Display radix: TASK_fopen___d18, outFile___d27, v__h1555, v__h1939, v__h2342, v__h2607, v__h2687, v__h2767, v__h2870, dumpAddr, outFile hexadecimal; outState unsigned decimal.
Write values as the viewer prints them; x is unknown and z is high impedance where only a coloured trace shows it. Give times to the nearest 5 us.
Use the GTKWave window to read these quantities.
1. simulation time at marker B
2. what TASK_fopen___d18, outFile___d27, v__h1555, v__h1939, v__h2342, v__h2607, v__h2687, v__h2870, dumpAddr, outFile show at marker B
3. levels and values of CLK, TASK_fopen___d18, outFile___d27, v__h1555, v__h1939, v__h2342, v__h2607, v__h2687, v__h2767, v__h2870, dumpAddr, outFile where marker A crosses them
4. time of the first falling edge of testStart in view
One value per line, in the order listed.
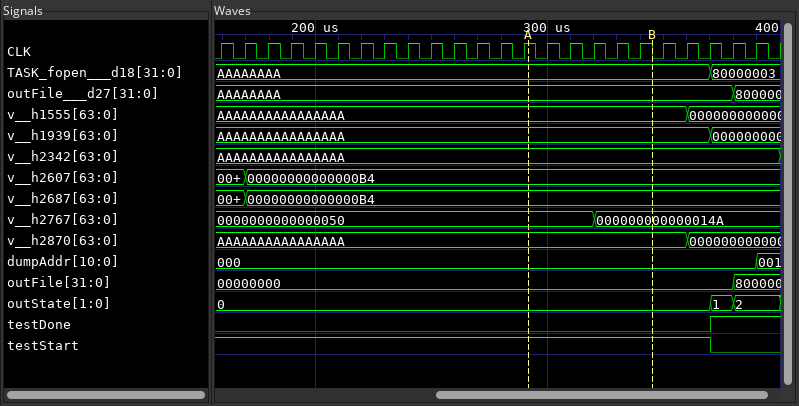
345 us
TASK_fopen___d18=AAAAAAAA, outFile___d27=AAAAAAAA, v__h1555=AAAAAAAAAAAAAAAA, v__h1939=AAAAAAAAAAAAAAAA, v__h2342=AAAAAAAAAAAAAAAA, v__h2607=00000000000000B4, v__h2687=00000000000000B4, v__h2870=AAAAAAAAAAAAAAAA, dumpAddr=000, outFile=00000000
CLK=1, TASK_fopen___d18=AAAAAAAA, outFile___d27=AAAAAAAA, v__h1555=AAAAAAAAAAAAAAAA, v__h1939=AAAAAAAAAAAAAAAA, v__h2342=AAAAAAAAAAAAAAAA, v__h2607=00000000000000B4, v__h2687=00000000000000B4, v__h2767=0000000000000050, v__h2870=AAAAAAAAAAAAAAAA, dumpAddr=000, outFile=00000000
370 us
